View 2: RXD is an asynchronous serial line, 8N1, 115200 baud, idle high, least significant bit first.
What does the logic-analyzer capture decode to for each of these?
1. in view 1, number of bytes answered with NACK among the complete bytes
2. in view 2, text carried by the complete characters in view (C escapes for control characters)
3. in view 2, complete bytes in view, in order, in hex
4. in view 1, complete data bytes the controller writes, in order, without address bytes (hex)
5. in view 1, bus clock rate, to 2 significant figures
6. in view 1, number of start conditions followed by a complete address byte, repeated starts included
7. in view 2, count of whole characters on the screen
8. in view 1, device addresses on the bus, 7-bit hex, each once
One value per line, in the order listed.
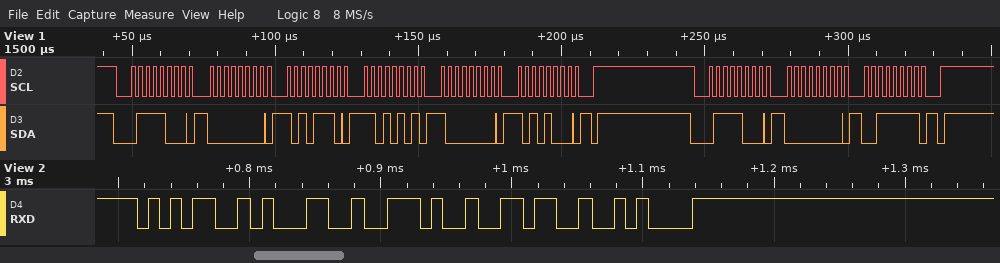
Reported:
0
"51.6\n"
35 31 2E 36 0A
00 AE D5 80 A8 00 3F
400 kHz
2
5
0x3C
